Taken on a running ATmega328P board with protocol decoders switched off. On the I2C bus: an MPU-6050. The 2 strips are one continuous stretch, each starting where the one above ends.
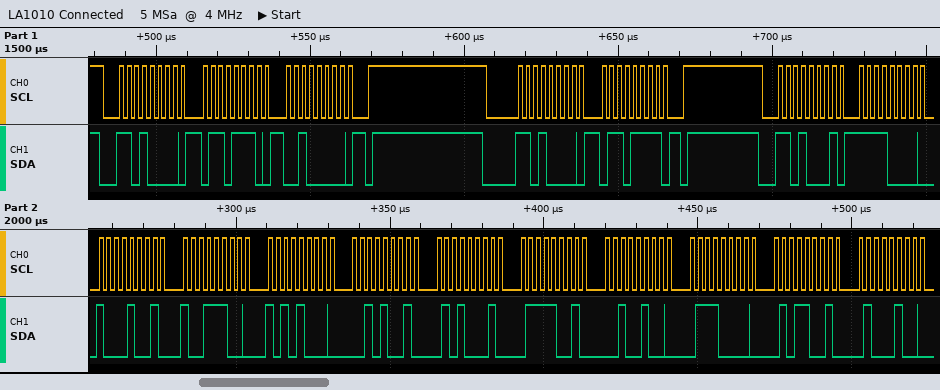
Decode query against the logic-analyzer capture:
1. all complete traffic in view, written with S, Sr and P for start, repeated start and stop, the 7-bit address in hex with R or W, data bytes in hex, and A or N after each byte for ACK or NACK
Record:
S 68W A 6E A 20 A P S 68W A 6F A P S 68R A F0 A 89 A 9C A A8 A 29 A 51 A 79 A 24 A 70 A 59 A 44 A
